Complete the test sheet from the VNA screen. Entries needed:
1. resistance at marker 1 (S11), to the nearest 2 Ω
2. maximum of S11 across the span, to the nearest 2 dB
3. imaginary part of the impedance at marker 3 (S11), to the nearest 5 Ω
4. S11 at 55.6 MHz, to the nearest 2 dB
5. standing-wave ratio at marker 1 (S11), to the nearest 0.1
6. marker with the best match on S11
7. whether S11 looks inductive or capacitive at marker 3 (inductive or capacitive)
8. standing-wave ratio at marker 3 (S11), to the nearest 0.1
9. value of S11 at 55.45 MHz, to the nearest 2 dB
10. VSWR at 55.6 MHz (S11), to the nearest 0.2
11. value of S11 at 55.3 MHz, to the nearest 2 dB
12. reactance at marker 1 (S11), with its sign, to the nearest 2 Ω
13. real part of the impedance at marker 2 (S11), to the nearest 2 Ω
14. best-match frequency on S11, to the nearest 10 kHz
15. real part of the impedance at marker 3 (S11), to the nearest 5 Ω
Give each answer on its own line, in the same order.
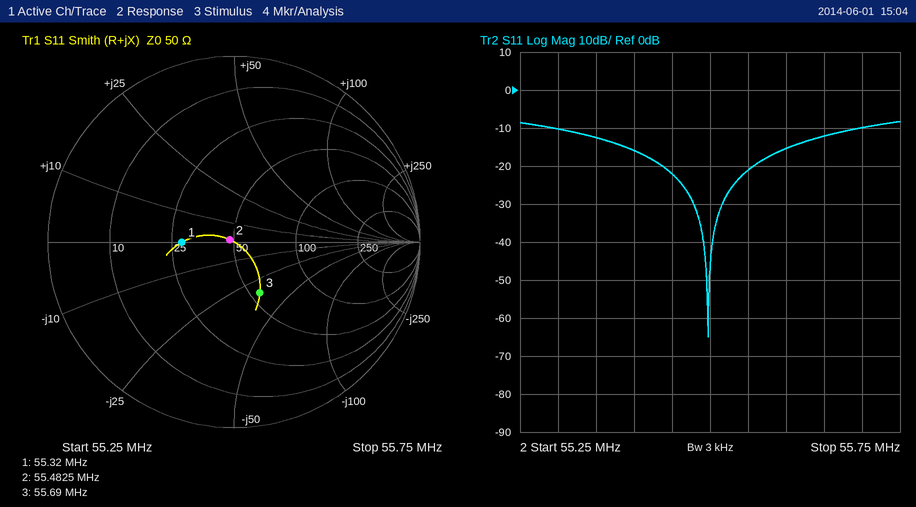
28 Ω
-8 dB
-35 Ω
-16 dB
1.8
marker 2
capacitive
1.9
-22 dB
1.4
-10 dB
0 Ω
48 Ω
55.50 MHz
55 Ω
